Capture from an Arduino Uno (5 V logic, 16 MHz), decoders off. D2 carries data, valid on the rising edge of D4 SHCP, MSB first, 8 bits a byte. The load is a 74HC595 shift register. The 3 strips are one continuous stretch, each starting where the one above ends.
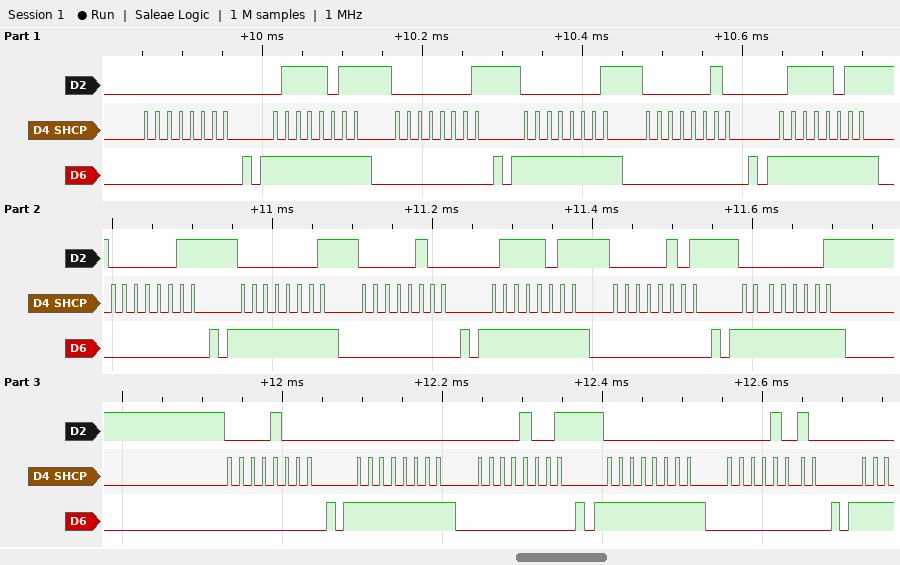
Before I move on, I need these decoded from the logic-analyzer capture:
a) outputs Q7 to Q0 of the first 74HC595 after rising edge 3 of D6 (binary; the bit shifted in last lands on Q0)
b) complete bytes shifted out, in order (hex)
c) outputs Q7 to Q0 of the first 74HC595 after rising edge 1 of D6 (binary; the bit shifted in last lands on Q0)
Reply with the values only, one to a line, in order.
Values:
00000001
0x00 0x7B 0x01 0x01 0x02 0x7B 0x03 0x01 0x04 0x7B 0x05 0x01 0x08 0x00 0x09 0x00 0x0A
00000000
